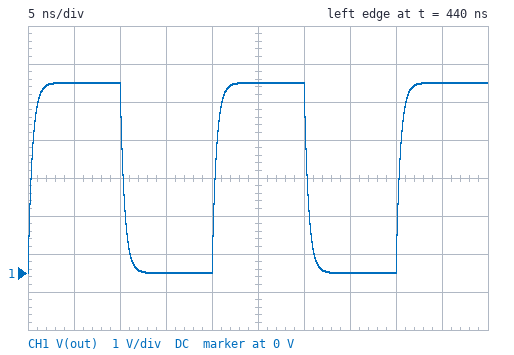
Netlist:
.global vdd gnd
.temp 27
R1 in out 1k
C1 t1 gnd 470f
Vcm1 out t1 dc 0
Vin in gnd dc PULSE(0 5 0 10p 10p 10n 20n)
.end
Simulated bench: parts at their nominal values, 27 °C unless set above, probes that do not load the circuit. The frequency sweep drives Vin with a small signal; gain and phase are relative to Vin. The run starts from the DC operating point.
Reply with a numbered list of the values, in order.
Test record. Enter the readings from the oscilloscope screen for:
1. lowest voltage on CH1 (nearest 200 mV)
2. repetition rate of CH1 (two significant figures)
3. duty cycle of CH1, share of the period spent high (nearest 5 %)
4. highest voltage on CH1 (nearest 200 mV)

1. 0 V
2. 50 MHz
3. 50 %
4. 5.0 V
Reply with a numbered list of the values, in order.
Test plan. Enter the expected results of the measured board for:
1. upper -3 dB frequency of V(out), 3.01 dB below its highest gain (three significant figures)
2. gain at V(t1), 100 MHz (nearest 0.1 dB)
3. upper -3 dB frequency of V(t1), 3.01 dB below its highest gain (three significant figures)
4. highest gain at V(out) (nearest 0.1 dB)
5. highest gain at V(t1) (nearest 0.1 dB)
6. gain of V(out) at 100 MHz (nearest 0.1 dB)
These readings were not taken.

1. 339 MHz
2. -0.4 dB
3. 339 MHz
4. 0 dB
5. 0 dB
6. -0.4 dB
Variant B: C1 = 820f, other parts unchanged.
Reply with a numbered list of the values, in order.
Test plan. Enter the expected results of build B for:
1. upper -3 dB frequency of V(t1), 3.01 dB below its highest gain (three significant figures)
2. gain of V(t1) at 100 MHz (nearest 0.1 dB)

1. 194 MHz
2. -1.0 dB
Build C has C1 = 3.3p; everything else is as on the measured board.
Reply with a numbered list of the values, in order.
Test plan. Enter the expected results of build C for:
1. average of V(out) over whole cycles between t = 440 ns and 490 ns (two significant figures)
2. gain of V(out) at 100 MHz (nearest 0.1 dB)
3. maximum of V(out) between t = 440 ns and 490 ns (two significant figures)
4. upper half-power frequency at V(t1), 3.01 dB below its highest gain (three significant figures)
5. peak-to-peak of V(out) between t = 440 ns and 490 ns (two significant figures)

1. 2.5 V
2. -7.2 dB
3. 4.8 V
4. 48.2 MHz
5. 4.5 V
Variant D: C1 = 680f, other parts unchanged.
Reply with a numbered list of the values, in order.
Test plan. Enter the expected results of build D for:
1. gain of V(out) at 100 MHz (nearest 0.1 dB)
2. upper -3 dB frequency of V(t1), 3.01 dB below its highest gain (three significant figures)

1. -0.7 dB
2. 234 MHz
